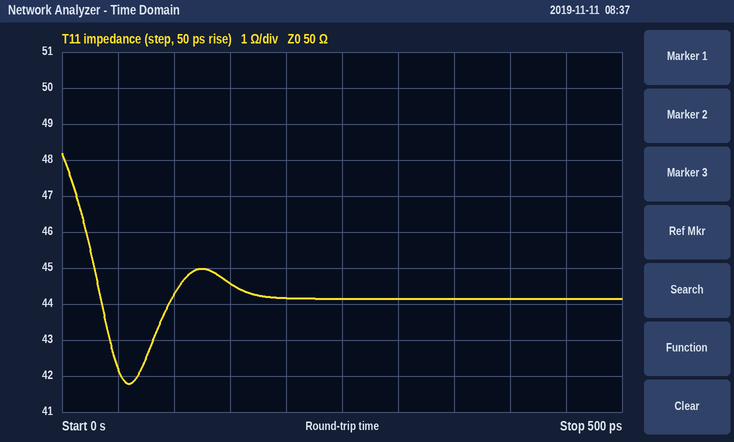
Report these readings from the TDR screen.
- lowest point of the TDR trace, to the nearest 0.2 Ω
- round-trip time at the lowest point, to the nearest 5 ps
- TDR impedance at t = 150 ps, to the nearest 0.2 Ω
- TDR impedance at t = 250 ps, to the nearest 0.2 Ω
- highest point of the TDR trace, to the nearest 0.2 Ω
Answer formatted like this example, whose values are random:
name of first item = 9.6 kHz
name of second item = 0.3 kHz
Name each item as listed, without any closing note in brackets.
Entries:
lowest point of the TDR trace, to the nearest 0.2 Ω = 41.8 Ω
round-trip time at the lowest point, to the nearest 5 ps = 60 ps
TDR impedance at t = 150 ps, to the nearest 0.2 Ω = 44.6 Ω
TDR impedance at t = 250 ps, to the nearest 0.2 Ω = 44.2 Ω
highest point of the TDR trace, to the nearest 0.2 Ω = 48.2 Ω
